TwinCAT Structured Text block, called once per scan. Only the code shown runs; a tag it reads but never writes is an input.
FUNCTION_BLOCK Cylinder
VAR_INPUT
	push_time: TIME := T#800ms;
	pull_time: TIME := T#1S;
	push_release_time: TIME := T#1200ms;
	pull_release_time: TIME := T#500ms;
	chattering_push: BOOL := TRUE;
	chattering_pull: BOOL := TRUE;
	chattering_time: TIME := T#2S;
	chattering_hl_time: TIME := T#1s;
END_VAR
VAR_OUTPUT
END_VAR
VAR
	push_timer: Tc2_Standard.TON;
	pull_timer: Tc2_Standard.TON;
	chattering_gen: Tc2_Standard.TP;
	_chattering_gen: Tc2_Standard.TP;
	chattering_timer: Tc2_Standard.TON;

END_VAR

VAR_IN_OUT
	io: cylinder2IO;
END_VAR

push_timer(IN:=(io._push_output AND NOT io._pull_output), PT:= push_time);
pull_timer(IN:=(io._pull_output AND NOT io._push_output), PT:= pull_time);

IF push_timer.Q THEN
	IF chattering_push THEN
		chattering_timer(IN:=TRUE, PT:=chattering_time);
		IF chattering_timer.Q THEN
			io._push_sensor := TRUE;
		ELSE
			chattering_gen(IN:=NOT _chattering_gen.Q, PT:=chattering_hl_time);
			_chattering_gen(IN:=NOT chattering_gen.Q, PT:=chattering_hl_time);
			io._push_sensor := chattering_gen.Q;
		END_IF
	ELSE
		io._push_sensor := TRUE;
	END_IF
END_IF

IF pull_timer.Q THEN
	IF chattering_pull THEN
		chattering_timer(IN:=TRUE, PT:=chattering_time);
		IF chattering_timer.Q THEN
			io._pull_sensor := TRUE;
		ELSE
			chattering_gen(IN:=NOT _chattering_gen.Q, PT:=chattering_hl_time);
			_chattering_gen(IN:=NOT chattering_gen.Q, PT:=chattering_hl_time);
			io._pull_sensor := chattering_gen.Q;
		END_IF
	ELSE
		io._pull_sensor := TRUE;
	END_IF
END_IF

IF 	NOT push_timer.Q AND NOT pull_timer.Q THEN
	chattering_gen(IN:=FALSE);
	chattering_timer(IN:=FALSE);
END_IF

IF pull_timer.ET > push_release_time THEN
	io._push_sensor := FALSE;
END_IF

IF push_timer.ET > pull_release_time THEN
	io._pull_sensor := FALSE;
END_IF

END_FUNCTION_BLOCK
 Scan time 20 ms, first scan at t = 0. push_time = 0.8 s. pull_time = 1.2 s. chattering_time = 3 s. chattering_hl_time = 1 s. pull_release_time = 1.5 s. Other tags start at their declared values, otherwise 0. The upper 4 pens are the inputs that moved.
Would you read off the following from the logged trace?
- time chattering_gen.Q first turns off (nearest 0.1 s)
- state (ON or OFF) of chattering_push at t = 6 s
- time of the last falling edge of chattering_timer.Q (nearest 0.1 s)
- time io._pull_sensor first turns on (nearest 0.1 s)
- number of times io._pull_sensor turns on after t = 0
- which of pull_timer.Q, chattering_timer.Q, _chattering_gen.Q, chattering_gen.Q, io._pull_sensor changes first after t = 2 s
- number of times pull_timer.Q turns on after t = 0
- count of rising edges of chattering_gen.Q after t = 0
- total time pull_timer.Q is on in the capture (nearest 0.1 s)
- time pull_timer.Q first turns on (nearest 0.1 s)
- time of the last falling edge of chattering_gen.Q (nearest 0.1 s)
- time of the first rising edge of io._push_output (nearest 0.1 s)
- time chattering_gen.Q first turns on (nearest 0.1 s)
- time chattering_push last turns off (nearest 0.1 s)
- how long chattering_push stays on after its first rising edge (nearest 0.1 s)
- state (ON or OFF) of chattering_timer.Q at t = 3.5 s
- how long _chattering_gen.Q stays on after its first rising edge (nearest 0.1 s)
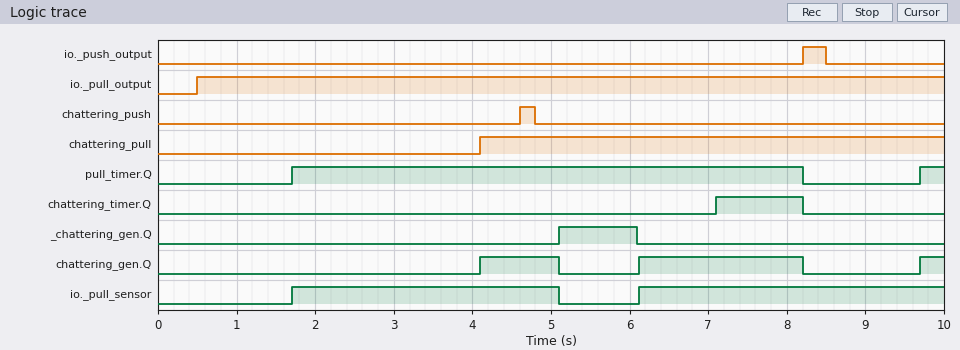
5.1 s
OFF
8.2 s
1.7 s
2
chattering_gen.Q
2
3
6.8 s
1.7 s
8.2 s
8.2 s
4.1 s
4.8 s
0.2 s
OFF
1.0 s
